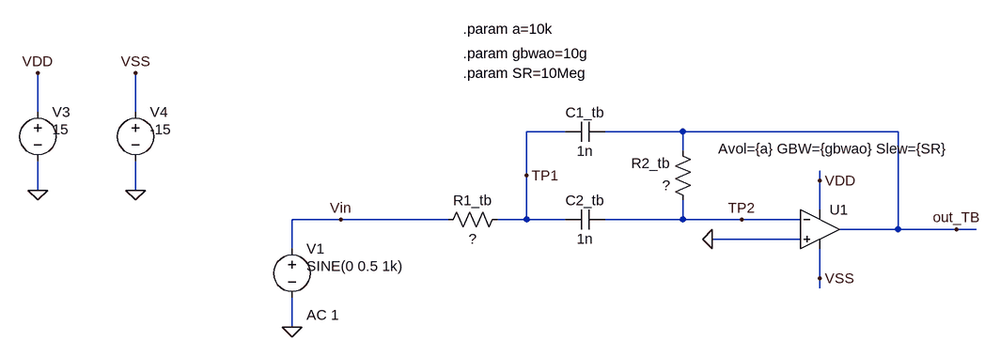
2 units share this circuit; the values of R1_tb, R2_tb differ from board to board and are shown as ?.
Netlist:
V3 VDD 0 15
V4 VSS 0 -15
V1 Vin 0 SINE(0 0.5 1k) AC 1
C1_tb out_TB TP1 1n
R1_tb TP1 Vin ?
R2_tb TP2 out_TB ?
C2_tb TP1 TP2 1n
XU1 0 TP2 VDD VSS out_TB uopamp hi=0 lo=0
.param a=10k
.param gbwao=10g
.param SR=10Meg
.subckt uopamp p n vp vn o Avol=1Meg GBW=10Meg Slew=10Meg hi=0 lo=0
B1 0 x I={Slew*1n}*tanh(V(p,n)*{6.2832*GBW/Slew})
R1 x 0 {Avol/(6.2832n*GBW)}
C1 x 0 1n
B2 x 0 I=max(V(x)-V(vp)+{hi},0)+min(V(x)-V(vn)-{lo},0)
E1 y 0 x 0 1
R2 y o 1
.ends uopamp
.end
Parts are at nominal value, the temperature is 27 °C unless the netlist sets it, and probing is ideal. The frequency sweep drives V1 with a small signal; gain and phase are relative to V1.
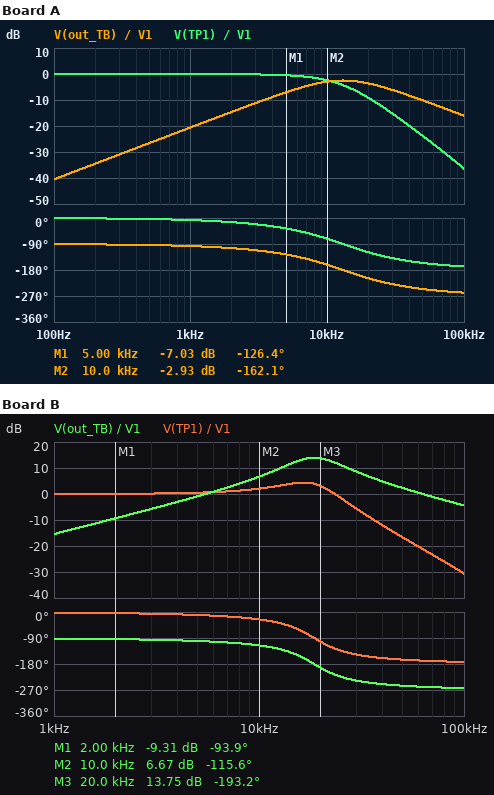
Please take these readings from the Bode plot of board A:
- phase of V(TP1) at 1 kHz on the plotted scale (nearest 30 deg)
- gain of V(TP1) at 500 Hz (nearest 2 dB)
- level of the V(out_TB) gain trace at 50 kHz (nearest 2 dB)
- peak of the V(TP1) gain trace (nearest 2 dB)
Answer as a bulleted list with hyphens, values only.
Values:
- 0 deg
- 0 dB
- -10 dB
- 0 dB
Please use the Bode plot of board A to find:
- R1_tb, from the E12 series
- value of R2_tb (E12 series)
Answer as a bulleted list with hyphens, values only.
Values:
- 10 kΩ
- 15 kΩ
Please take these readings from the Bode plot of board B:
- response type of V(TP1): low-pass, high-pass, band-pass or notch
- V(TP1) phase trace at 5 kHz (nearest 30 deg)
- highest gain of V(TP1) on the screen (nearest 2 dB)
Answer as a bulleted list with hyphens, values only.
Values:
- low-pass
- 0 deg
- 4 dB
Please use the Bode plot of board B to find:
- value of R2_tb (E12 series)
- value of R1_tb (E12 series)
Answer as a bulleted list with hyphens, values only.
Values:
- 27 kΩ
- 2.7 kΩ
